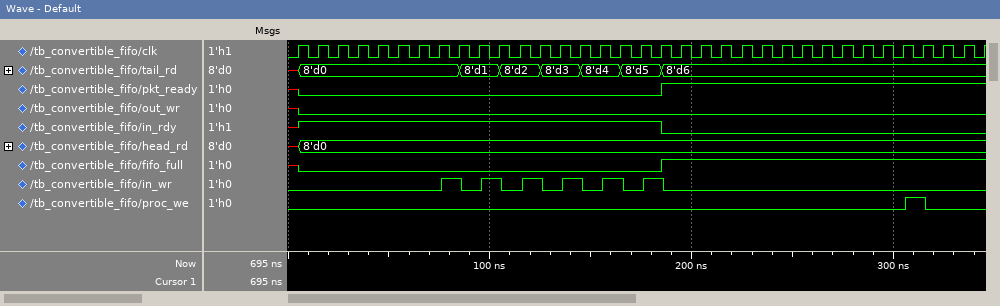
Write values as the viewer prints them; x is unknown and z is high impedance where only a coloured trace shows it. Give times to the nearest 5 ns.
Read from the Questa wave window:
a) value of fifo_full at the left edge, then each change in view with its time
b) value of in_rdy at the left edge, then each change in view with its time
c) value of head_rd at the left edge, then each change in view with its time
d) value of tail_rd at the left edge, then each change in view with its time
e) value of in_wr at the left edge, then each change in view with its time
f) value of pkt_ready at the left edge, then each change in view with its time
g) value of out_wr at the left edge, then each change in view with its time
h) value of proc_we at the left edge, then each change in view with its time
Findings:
x, 0 at 5 ns, 1 at 185 ns
x, 1 at 5 ns, 0 at 185 ns
x, 8'd0 at 5 ns
x, 8'd0 at 5 ns, 8'd1 at 85 ns, 8'd2 at 105 ns, 8'd3 at 125 ns, 8'd4 at 145 ns, 8'd5 at 165 ns, 8'd6 at 185 ns
0, 1 at 75 ns, 0 at 85 ns, 1 at 95 ns, 0 at 105 ns, 1 at 115 ns, 0 at 125 ns, 1 at 135 ns, 0 at 145 ns, 1 at 155 ns, 0 at 165 ns, 1 at 175 ns, 0 at 185 ns
x, 0 at 5 ns, 1 at 185 ns
x, 0 at 5 ns
0, 1 at 305 ns, 0 at 315 ns
